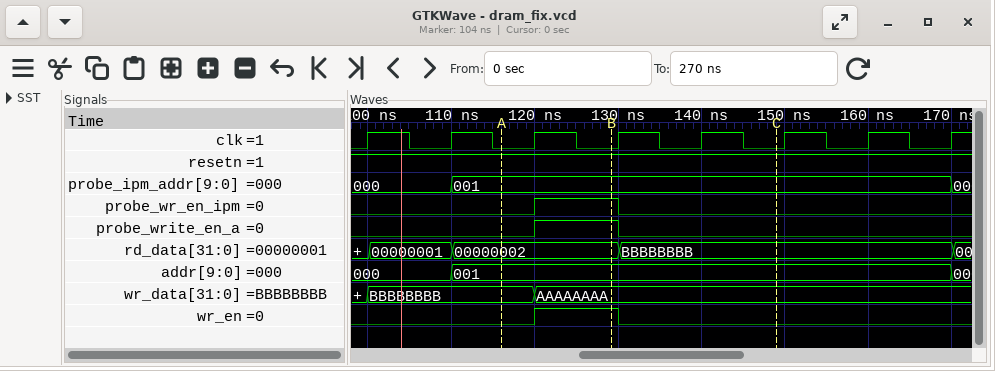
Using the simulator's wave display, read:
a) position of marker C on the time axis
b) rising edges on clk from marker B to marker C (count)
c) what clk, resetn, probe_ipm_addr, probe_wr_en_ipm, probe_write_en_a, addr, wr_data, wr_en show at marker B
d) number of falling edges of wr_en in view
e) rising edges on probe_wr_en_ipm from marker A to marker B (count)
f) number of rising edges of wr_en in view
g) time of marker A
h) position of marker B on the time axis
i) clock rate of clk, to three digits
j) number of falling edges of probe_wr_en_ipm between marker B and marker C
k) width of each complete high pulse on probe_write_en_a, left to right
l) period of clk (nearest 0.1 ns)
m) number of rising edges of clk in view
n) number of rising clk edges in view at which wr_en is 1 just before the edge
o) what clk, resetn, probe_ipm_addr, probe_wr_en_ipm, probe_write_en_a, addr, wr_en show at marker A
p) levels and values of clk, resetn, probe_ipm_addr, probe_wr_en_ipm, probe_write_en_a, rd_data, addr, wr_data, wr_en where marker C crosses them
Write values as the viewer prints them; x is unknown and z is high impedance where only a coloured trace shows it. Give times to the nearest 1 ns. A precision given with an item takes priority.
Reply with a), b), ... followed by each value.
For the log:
a) 149 ns
b) 2
c) clk=0, resetn=1, probe_ipm_addr=001, probe_wr_en_ipm=1, probe_write_en_a=1, addr=001, wr_data=AAAAAAAA, wr_en=1
d) 1
e) 1
f) 1
g) 116 ns
h) 129 ns
i) 100 MHz
j) 1
k) 10 ns
l) 10 ns
m) 8
n) 1
o) clk=0, resetn=1, probe_ipm_addr=001, probe_wr_en_ipm=0, probe_write_en_a=0, addr=001, wr_en=0
p) clk=0, resetn=1, probe_ipm_addr=001, probe_wr_en_ipm=0, probe_write_en_a=0, rd_data=BBBBBBBB, addr=001, wr_data=AAAAAAAA, wr_en=0
